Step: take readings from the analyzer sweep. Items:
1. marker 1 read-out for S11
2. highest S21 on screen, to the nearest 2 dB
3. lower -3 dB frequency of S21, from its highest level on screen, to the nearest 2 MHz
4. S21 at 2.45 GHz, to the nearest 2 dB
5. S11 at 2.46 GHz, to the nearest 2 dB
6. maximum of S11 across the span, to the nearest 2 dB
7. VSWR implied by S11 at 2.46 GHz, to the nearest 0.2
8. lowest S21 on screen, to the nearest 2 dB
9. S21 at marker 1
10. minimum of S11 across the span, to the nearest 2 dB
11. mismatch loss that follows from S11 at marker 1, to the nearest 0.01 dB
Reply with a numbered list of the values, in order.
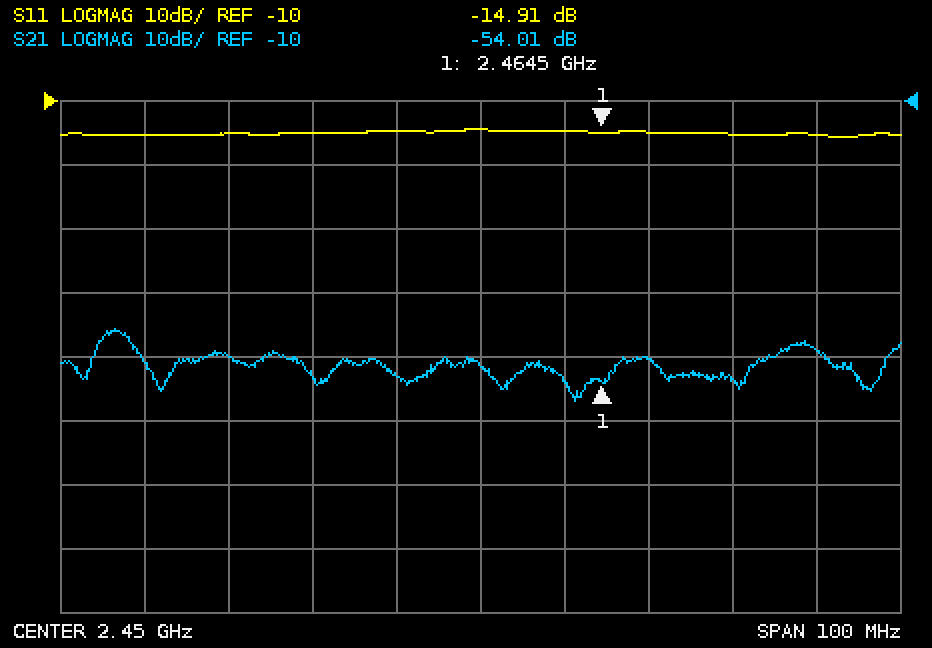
1. -14.91 dB
2. -46 dB
3. 2.404 GHz
4. -52 dB
5. -14 dB
6. -14 dB
7. 1.4
8. -56 dB
9. -54.01 dB
10. -16 dB
11. 0.14 dB
